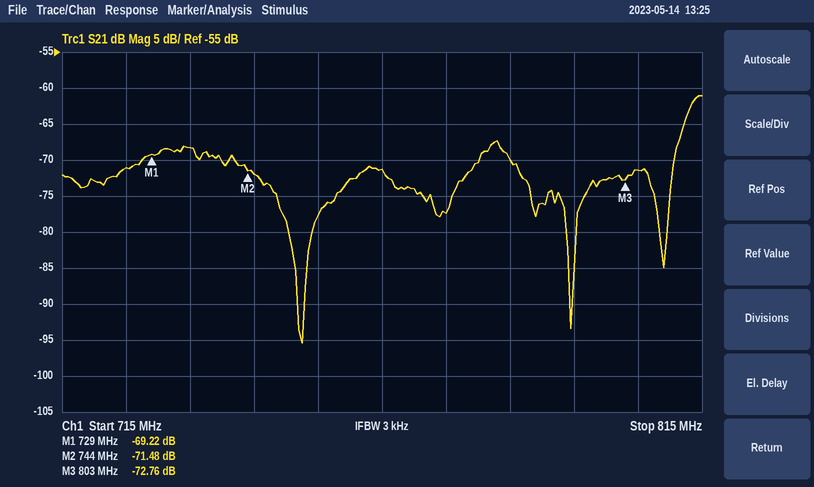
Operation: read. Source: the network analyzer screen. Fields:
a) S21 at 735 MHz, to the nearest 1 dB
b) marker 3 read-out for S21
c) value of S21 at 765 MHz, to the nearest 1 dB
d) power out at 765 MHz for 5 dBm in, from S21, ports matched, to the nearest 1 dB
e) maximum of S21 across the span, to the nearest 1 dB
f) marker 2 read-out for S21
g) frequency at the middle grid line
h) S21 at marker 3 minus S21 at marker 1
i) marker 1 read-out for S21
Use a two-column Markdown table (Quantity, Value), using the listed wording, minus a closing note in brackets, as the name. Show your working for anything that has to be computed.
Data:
| Quantity | Value |
|---|---|
| S21 at 735 MHz, to the nearest 1 dB | -68 dB |
| marker 3 read-out for S21 | -72.76 dB |
| value of S21 at 765 MHz, to the nearest 1 dB | -71 dB |
| power out at 765 MHz for 5 dBm in, from S21, ports matched, to the nearest 1 dB | 5 dBm + (-71 dB) = -66 dBm |
| maximum of S21 across the span, to the nearest 1 dB | -61 dB |
| marker 2 read-out for S21 | -71.48 dB |
| frequency at the middle grid line | 765 MHz |
| S21 at marker 3 minus S21 at marker 1 | -72.76 − (-69.22) = -3.54 dB |
| marker 1 read-out for S21 | -69.22 dB |
